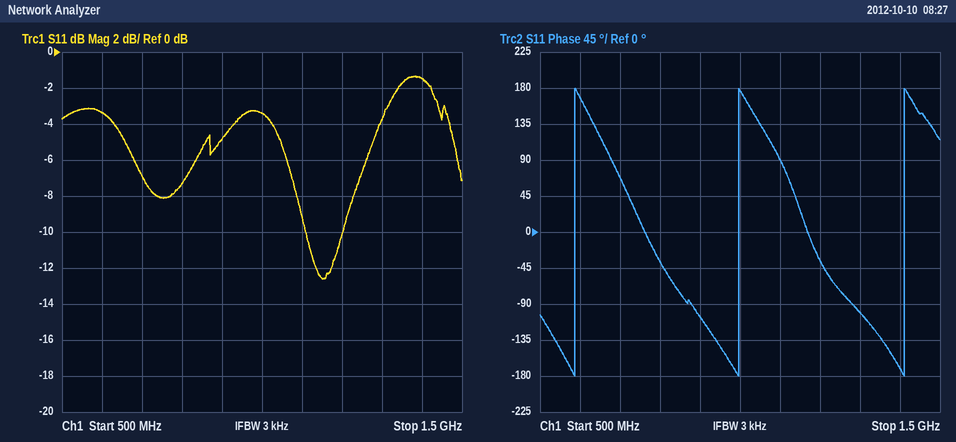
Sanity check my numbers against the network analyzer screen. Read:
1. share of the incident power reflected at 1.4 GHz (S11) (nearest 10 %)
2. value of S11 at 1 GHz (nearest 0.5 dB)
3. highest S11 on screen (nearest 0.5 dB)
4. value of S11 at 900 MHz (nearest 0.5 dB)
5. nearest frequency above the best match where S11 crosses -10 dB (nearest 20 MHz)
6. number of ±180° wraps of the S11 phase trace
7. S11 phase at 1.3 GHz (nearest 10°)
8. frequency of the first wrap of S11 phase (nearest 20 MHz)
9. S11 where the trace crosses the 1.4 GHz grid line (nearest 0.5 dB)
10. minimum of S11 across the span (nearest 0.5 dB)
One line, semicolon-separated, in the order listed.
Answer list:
70 %; -3.5 dB; -1.5 dB; -5.0 dB; 1.20 GHz; 3; -100°; 580 MHz; -1.5 dB; -12.5 dB
